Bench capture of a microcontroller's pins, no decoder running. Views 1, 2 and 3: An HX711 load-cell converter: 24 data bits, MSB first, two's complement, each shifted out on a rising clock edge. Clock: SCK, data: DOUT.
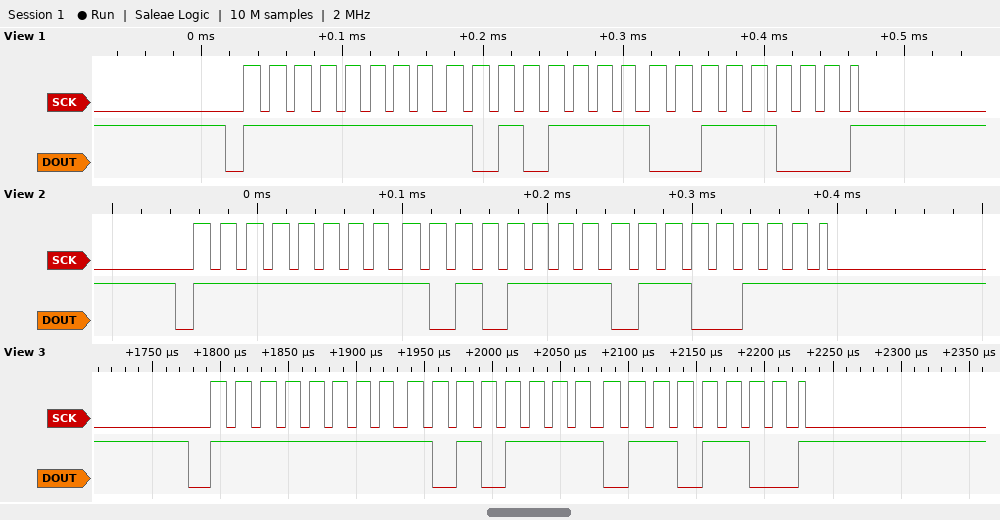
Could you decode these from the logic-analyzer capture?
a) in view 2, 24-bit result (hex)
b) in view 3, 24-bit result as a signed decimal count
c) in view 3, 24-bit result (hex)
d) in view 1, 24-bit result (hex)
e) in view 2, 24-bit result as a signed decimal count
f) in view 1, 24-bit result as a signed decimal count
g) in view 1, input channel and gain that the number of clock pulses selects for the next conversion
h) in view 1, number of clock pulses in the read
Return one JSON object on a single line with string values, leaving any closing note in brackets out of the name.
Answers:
{"in view 2, 24-bit result": "0xFFAF67", "in view 3, 24-bit result as a signed decimal count": "-20628", "in view 3, 24-bit result": "0xFFAF6C", "in view 1, 24-bit result": "0xFFAF38", "in view 2, 24-bit result as a signed decimal count": "-20633", "in view 1, 24-bit result as a signed decimal count": "-20680", "in view 1, input channel and gain that the number of clock pulses selects for the next conversion": "channel A, gain 128", "in view 1, number of clock pulses in the read": "25"}
